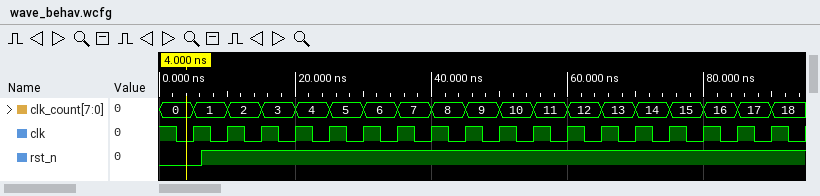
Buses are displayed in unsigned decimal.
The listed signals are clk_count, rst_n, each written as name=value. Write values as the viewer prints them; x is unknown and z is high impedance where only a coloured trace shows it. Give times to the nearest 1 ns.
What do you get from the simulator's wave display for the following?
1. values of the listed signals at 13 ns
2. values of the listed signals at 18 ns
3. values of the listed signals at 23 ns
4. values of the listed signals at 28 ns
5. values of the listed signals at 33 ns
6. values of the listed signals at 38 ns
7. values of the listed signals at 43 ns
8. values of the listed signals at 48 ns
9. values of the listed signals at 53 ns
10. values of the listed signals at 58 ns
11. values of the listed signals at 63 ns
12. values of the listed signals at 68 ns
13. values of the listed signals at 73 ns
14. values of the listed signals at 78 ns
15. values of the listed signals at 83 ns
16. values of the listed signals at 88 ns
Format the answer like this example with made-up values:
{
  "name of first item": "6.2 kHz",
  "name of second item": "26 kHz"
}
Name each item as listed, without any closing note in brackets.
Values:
{
  "values of the listed signals at 13 ns": "clk_count=2, rst_n=1",
  "values of the listed signals at 18 ns": "clk_count=3, rst_n=1",
  "values of the listed signals at 23 ns": "clk_count=4, rst_n=1",
  "values of the listed signals at 28 ns": "clk_count=5, rst_n=1",
  "values of the listed signals at 33 ns": "clk_count=6, rst_n=1",
  "values of the listed signals at 38 ns": "clk_count=7, rst_n=1",
  "values of the listed signals at 43 ns": "clk_count=8, rst_n=1",
  "values of the listed signals at 48 ns": "clk_count=9, rst_n=1",
  "values of the listed signals at 53 ns": "clk_count=10, rst_n=1",
  "values of the listed signals at 58 ns": "clk_count=11, rst_n=1",
  "values of the listed signals at 63 ns": "clk_count=12, rst_n=1",
  "values of the listed signals at 68 ns": "clk_count=13, rst_n=1",
  "values of the listed signals at 73 ns": "clk_count=14, rst_n=1",
  "values of the listed signals at 78 ns": "clk_count=15, rst_n=1",
  "values of the listed signals at 83 ns": "clk_count=16, rst_n=1",
  "values of the listed signals at 88 ns": "clk_count=17, rst_n=1"
}
